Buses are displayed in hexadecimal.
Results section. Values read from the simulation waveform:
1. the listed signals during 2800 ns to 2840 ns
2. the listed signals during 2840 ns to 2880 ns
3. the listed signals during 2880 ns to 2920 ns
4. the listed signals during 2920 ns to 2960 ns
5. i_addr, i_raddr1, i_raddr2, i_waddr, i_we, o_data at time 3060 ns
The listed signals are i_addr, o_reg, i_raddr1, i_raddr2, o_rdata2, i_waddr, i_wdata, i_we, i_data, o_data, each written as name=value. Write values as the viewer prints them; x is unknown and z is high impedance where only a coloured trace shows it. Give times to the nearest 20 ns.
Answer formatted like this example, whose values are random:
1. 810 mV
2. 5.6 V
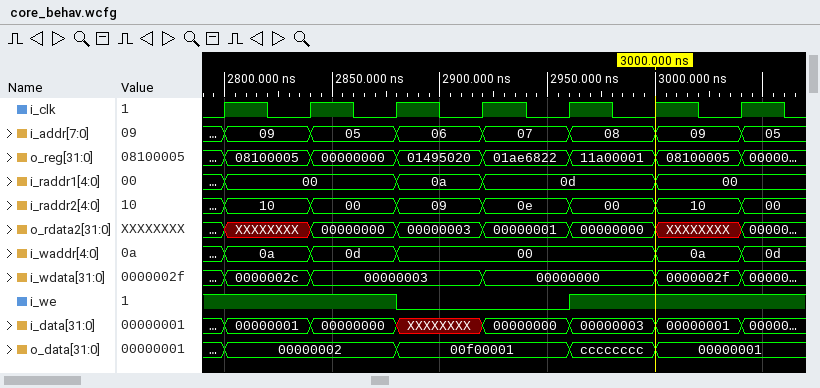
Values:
1. i_addr=09, o_reg=08100005, i_raddr1=00, i_raddr2=10, o_rdata2=XXXXXXXX, i_waddr=0a, i_wdata=0000002c, i_we=1, i_data=00000001, o_data=00000002
2. i_addr=05, o_reg=00000000, i_raddr1=00, i_raddr2=00, o_rdata2=00000000, i_waddr=0d, i_wdata=00000003, i_we=1, i_data=00000000, o_data=00000002
3. i_addr=06, o_reg=01495020, i_raddr1=0a, i_raddr2=09, o_rdata2=00000003, i_waddr=00, i_wdata=00000003, i_we=0, i_data=XXXXXXXX, o_data=00f00001
4. i_addr=07, o_reg=01ae6822, i_raddr1=0d, i_raddr2=0e, o_rdata2=00000001, i_waddr=00, i_wdata=00000000, i_we=0, i_data=00000000, o_data=00f00001
5. i_addr=05, i_raddr1=00, i_raddr2=00, i_waddr=0d, i_we=1, o_data=00000001
